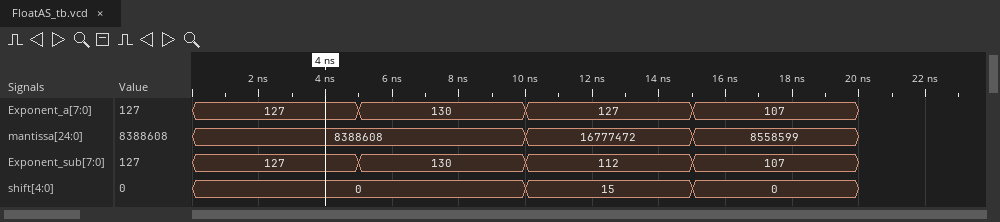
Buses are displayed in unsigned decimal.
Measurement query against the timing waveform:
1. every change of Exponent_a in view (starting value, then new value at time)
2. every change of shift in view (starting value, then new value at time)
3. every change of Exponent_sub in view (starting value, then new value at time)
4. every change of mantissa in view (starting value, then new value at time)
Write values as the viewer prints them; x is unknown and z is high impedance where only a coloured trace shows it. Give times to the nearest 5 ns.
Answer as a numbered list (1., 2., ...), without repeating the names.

1. 127, 130 at 5 ns, 127 at 10 ns, 107 at 15 ns
2. 0, 15 at 10 ns, 0 at 15 ns
3. 127, 130 at 5 ns, 112 at 10 ns, 107 at 15 ns
4. 8388608, 16777472 at 10 ns, 8558599 at 15 ns
